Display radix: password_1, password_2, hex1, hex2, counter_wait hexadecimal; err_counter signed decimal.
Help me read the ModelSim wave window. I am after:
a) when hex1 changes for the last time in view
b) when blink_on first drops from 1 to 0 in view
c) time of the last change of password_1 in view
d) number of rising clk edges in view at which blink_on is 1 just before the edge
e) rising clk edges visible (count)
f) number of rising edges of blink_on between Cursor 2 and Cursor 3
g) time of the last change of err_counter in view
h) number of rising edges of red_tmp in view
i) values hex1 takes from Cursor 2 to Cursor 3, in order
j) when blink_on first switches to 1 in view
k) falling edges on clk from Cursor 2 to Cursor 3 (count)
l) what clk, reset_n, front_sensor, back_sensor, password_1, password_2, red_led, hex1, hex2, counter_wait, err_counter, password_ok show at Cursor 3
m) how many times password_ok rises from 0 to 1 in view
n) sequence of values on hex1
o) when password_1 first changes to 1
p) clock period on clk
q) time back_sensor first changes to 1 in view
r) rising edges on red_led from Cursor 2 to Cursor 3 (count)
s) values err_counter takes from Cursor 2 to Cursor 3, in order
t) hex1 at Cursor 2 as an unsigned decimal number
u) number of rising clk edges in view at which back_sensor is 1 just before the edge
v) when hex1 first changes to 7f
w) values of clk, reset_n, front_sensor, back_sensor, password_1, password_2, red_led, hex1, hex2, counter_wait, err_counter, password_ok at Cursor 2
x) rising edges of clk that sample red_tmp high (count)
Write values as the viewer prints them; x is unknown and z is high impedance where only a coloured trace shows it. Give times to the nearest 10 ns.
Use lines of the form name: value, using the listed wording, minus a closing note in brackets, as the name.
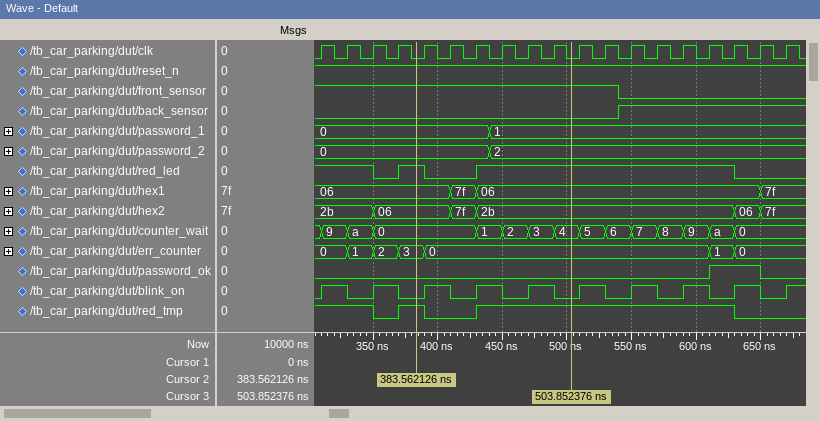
when hex1 changes for the last time in view: 650 ns
when blink_on first drops from 1 to 0 in view: 330 ns
time of the last change of password_1 in view: 440 ns
number of rising clk edges in view at which blink_on is 1 just before the edge: 9
rising clk edges visible: 19
number of rising edges of blink_on between Cursor 2 and Cursor 3: 3
time of the last change of err_counter in view: 630 ns
number of rising edges of red_tmp in view: 2
values hex1 takes from Cursor 2 to Cursor 3, in order: 06, 7f, 06
when blink_on first switches to 1 in view: 310 ns
falling edges on clk from Cursor 2 to Cursor 3: 6
what clk, reset_n, front_sensor, back_sensor, password_1, password_2, red_led, hex1, hex2, counter_wait, err_counter, password_ok show at Cursor 3: clk=0, reset_n=1, front_sensor=1, back_sensor=0, password_1=1, password_2=2, red_led=1, hex1=06, hex2=2b, counter_wait=4, err_counter=0, password_ok=0
how many times password_ok rises from 0 to 1 in view: 1
sequence of values on hex1: 06, 7f, 06, 7f
when password_1 first changes to 1: 440 ns
clock period on clk: 20 ns
time back_sensor first changes to 1 in view: 540 ns
rising edges on red_led from Cursor 2 to Cursor 3: 1
values err_counter takes from Cursor 2 to Cursor 3, in order: 3, 0
hex1 at Cursor 2 as an unsigned decimal number: 6
number of rising clk edges in view at which back_sensor is 1 just before the edge: 7
when hex1 first changes to 7f: 410 ns
values of clk, reset_n, front_sensor, back_sensor, password_1, password_2, red_led, hex1, hex2, counter_wait, err_counter, password_ok at Cursor 2: clk=0, reset_n=1, front_sensor=1, back_sensor=0, password_1=0, password_2=0, red_led=1, hex1=06, hex2=06, counter_wait=0, err_counter=3, password_ok=0
rising edges of clk that sample red_tmp high: 14
